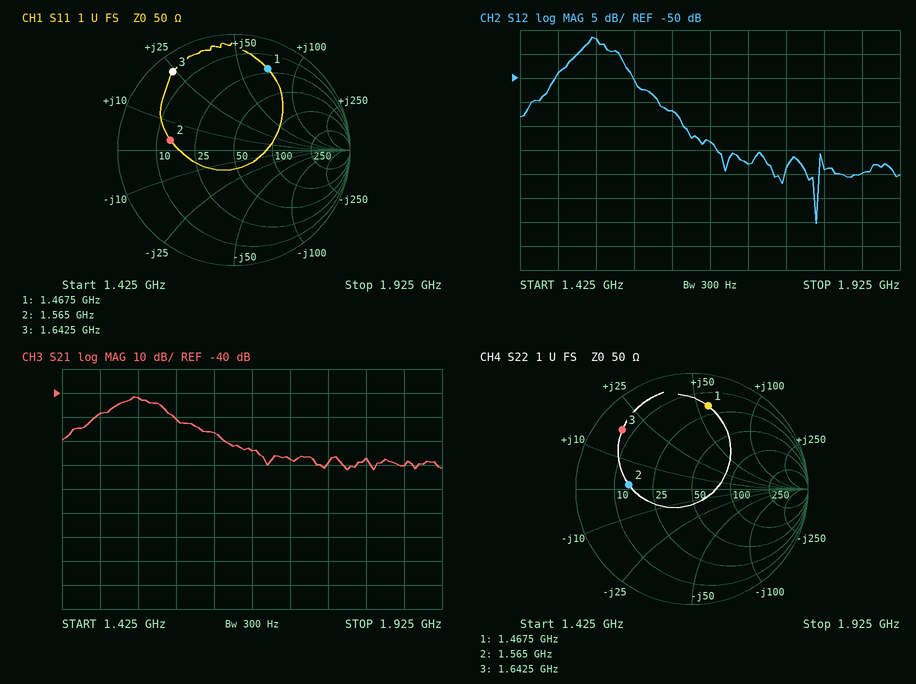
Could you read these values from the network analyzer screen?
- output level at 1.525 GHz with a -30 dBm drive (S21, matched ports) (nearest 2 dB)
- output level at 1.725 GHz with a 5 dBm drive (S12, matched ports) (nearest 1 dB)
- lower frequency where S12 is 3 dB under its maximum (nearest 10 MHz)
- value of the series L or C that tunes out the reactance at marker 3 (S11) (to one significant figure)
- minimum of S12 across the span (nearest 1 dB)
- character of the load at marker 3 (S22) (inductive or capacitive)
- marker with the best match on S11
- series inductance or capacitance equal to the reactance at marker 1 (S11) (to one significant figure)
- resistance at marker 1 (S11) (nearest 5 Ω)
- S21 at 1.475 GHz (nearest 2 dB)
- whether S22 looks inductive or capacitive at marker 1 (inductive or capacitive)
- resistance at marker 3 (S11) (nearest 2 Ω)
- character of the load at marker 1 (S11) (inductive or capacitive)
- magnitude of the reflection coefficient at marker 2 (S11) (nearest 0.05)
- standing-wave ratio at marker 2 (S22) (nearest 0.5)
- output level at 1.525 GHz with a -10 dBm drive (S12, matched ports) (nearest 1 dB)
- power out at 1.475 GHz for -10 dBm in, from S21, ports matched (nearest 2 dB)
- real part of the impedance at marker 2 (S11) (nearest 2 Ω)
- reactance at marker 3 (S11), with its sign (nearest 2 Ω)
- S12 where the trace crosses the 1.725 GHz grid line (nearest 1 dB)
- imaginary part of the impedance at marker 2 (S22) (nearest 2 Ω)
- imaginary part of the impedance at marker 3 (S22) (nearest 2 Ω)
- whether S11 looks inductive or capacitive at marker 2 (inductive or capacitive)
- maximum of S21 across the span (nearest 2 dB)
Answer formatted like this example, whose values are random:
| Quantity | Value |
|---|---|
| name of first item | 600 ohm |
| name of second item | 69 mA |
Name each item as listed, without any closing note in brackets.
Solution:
| Quantity | Value |
|---|---|
| output level at 1.525 GHz with a -30 dBm drive (S21, matched ports) | -72 dBm |
| output level at 1.725 GHz with a 5 dBm drive (S12, matched ports) | -63 dBm |
| lower frequency where S12 is 3 dB under its maximum | 1.50 GHz |
| value of the series L or C that tunes out the reactance at marker 3 (S11) | 4 pF |
| minimum of S12 across the span | -80 dB |
| character of the load at marker 3 (S22) | inductive |
| marker with the best match on S11 | marker 2 |
| series inductance or capacitance equal to the reactance at marker 1 (S11) | 8 nH |
| resistance at marker 1 (S11) | 20 Ω |
| S21 at 1.475 GHz | -48 dB |
| whether S22 looks inductive or capacitive at marker 1 | inductive |
| resistance at marker 3 (S11) | 4 Ω |
| character of the load at marker 1 (S11) | inductive |
| magnitude of the reflection coefficient at marker 2 (S11) | 0.55 |
| standing-wave ratio at marker 2 (S22) | 3.5 |
| output level at 1.525 GHz with a -10 dBm drive (S12, matched ports) | -52 dBm |
| power out at 1.475 GHz for -10 dBm in, from S21, ports matched | -58 dBm |
| real part of the impedance at marker 2 (S11) | 14 Ω |
| reactance at marker 3 (S11), with its sign | +24 Ω |
| S12 where the trace crosses the 1.725 GHz grid line | -68 dB |
| imaginary part of the impedance at marker 2 (S22) | +2 Ω |
| imaginary part of the impedance at marker 3 (S22) | +18 Ω |
| whether S11 looks inductive or capacitive at marker 2 | inductive |
| maximum of S21 across the span | -42 dB |
